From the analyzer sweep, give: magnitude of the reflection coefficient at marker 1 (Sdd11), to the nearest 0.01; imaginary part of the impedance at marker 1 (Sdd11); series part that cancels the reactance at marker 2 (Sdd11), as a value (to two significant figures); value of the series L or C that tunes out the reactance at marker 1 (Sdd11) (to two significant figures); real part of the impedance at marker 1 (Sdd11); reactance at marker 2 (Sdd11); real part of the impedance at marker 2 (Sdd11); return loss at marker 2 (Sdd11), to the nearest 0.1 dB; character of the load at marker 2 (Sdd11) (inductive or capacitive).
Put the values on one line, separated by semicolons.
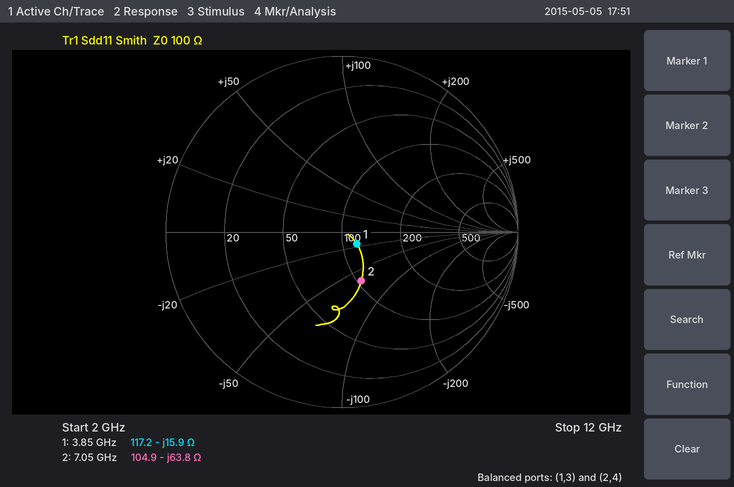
0.11; -15.9 Ω; 1.4 nH; 660 pH; 117.2 Ω; -63.8 Ω; 104.9 Ω; 10.5 dB; capacitive
